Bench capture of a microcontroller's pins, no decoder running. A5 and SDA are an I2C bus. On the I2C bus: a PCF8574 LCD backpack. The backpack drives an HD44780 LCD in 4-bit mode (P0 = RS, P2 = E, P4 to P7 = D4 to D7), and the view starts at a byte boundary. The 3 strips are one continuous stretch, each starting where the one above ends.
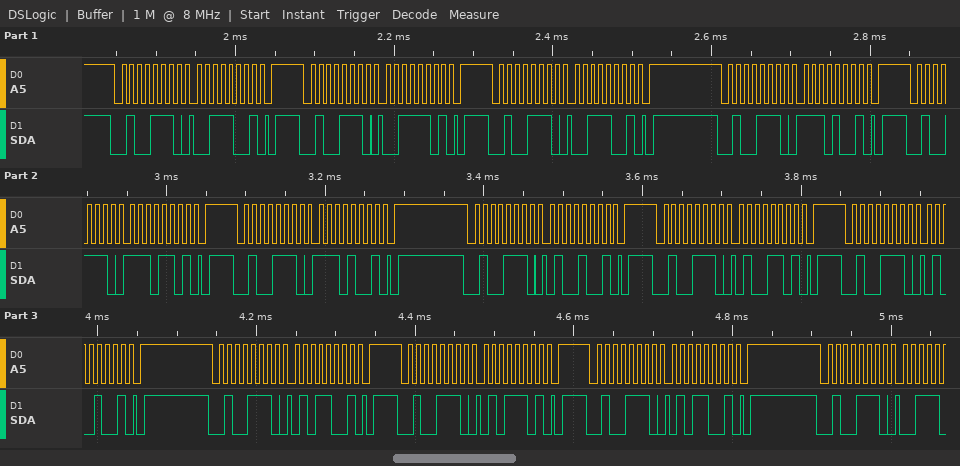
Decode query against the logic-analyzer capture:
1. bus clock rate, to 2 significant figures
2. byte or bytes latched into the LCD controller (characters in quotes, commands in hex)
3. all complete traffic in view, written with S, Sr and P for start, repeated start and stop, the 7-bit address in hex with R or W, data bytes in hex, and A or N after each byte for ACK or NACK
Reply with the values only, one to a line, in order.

100 kHz
'>' 'E'
S 27W A 39 A P S 27W A 3D A P S 27W A 39 A P S 27W A E9 A P S 27W A ED A P S 27W A E9 A P S 27W A 49 A P S 27W A 4D A P S 27W A 49 A P S 27W A 59 A P S 27W A 5D A P S 27W A 59 A P S 27W A
